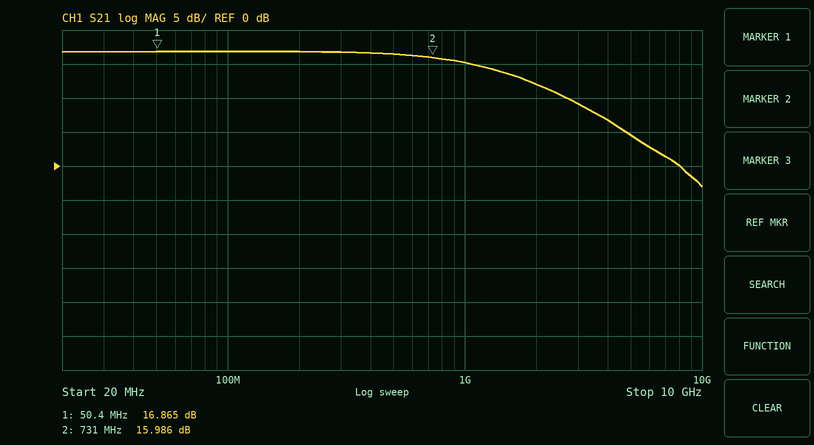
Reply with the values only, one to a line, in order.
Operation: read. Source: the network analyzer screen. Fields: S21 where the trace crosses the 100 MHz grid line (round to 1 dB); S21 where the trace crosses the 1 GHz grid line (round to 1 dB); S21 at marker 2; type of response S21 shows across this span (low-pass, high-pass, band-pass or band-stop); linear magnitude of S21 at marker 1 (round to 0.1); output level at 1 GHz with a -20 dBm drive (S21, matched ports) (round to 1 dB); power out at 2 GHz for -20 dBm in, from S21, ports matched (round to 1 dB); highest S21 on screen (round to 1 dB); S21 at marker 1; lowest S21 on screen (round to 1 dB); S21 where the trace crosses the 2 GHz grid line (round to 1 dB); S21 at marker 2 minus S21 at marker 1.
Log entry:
17 dB
15 dB
15.986 dB
low-pass
7.0
-5 dBm
-8 dBm
17 dB
16.865 dB
-3 dB
12 dB
-0.879 dB
